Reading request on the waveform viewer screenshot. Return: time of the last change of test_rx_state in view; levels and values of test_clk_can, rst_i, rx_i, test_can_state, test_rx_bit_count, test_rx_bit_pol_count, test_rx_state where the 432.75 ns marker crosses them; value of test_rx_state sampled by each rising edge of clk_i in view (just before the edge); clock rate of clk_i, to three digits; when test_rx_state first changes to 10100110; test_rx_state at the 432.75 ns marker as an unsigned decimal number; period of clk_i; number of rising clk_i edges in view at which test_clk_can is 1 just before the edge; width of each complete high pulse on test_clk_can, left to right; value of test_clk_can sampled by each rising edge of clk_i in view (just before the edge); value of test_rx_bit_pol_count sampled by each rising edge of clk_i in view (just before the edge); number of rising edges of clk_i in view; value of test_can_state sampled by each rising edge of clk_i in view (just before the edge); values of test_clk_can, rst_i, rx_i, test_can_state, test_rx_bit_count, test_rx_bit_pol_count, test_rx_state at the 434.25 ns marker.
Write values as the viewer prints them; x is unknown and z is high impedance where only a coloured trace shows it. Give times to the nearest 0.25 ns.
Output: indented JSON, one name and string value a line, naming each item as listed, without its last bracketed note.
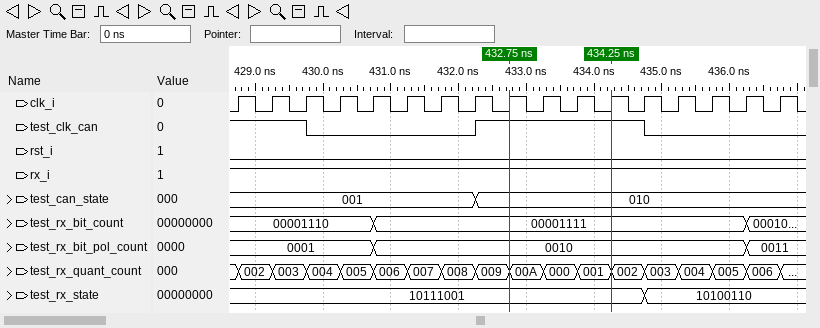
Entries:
{
  "time of the last change of test_rx_state in view": "434.75 ns",
  "levels and values of test_clk_can, rst_i, rx_i, test_can_state, test_rx_bit_count, test_rx_bit_pol_count, test_rx_state where the 432.75 ns marker crosses them": "test_clk_can=1, rst_i=0, rx_i=1, test_can_state=010, test_rx_bit_count=00001111, test_rx_bit_pol_count=0010, test_rx_state=10111001",
  "value of test_rx_state sampled by each rising edge of clk_i in view": "10111001, 10111001, 10111001, 10111001, 10111001, 10111001, 10111001, 10111001, 10111001, 10111001, 10111001, 10111001, 10111001, 10100110, 10100110, 10100110, 10100110",
  "clock rate of clk_i, to three digits": "2.00 GHz",
  "when test_rx_state first changes to 10100110": "434.75 ns",
  "test_rx_state at the 432.75 ns marker as an unsigned decimal number": "185",
  "period of clk_i": "0.5 ns",
  "number of rising clk_i edges in view at which test_clk_can is 1 just before the edge": "8",
  "width of each complete high pulse on test_clk_can, left to right": "2.5 ns",
  "value of test_clk_can sampled by each rising edge of clk_i in view": "1 1 1 0 0 0 0 0 1 1 1 1 1 0 0 0 0",
  "value of test_rx_bit_pol_count sampled by each rising edge of clk_i in view": "0001, 0001, 0001, 0001, 0001, 0010, 0010, 0010, 0010, 0010, 0010, 0010, 0010, 0010, 0010, 0010, 0011",
  "number of rising edges of clk_i in view": "17",
  "value of test_can_state sampled by each rising edge of clk_i in view": "001, 001, 001, 001, 001, 001, 001, 001, 010, 010, 010, 010, 010, 010, 010, 010, 010",
  "values of test_clk_can, rst_i, rx_i, test_can_state, test_rx_bit_count, test_rx_bit_pol_count, test_rx_state at the 434.25 ns marker": "test_clk_can=1, rst_i=0, rx_i=1, test_can_state=010, test_rx_bit_count=00001111, test_rx_bit_pol_count=0010, test_rx_state=10111001"
}
